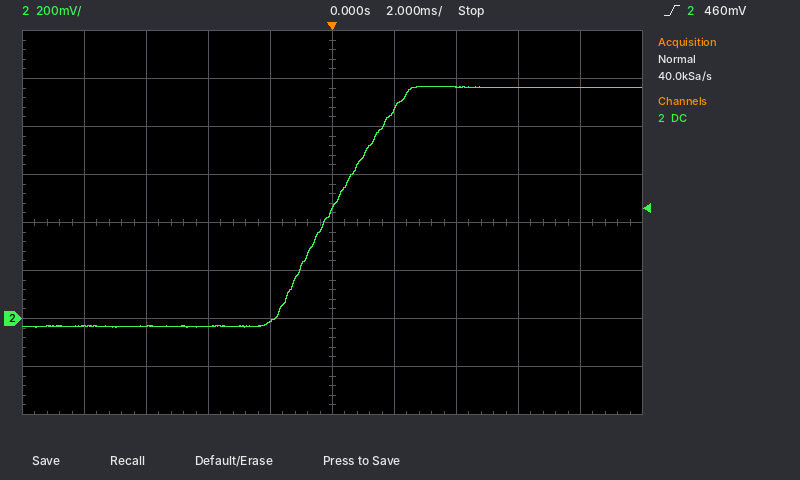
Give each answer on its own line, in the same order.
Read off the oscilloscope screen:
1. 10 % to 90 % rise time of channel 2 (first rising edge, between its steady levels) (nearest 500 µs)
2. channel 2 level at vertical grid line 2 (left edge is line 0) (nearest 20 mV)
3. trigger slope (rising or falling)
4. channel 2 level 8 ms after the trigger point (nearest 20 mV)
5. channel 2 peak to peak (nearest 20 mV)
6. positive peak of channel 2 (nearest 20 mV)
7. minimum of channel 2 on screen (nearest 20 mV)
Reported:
3.5 ms
-40 mV
rising
960 mV
1.00 V
960 mV
-40 mV
